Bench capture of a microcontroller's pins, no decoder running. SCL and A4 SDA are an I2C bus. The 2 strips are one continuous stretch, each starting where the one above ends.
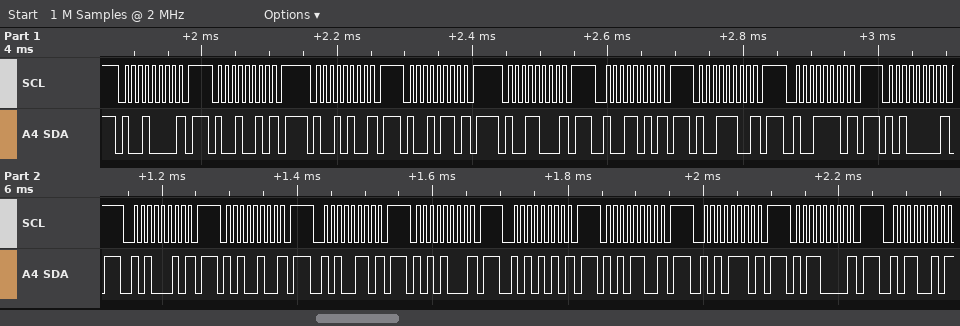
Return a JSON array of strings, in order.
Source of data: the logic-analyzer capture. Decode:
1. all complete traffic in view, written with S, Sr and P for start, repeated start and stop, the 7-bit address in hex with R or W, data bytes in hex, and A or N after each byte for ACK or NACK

["S 48W N P S 49W N P S 4AW N P S 4BW N P S 4CW N P S 4DW N P S 4EW N P S 4FW N P S 50W N P S 51W N P S 52W N P S 53W N P S 54W N P S 55W N P S 56W N P S 57W N P S 58W N P S 59W N"]
